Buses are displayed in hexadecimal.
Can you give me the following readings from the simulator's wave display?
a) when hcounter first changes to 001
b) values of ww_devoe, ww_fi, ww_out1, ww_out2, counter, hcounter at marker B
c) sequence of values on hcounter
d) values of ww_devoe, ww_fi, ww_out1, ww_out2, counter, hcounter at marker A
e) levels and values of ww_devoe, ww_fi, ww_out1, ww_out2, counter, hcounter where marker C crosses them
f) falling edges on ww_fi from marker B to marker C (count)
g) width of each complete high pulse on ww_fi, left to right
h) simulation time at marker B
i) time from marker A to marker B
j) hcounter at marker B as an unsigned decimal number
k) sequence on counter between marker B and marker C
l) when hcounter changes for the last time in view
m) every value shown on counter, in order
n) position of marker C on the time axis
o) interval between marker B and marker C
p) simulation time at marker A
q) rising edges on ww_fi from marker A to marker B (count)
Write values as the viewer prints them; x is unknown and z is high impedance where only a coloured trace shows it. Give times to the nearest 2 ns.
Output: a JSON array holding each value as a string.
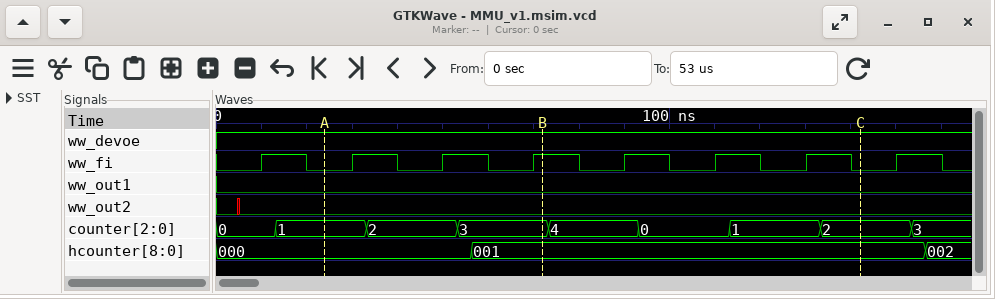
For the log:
["56 ns", "ww_devoe=1, ww_fi=1, ww_out1=0, ww_out2=0, counter=3, hcounter=001", "000, 001, 002", "ww_devoe=1, ww_fi=0, ww_out1=0, ww_out2=0, counter=1, hcounter=000", "ww_devoe=1, ww_fi=0, ww_out1=0, ww_out2=0, counter=2, hcounter=001", "4", "10 ns, 10 ns, 10 ns, 10 ns, 10 ns, 10 ns, 10 ns, 10 ns", "72 ns", "48 ns", "1", "3, 4, 0, 1, 2", "156 ns", "0, 1, 2, 3, 4, 0, 1, 2, 3", "142 ns", "70 ns", "24 ns", "3"]
